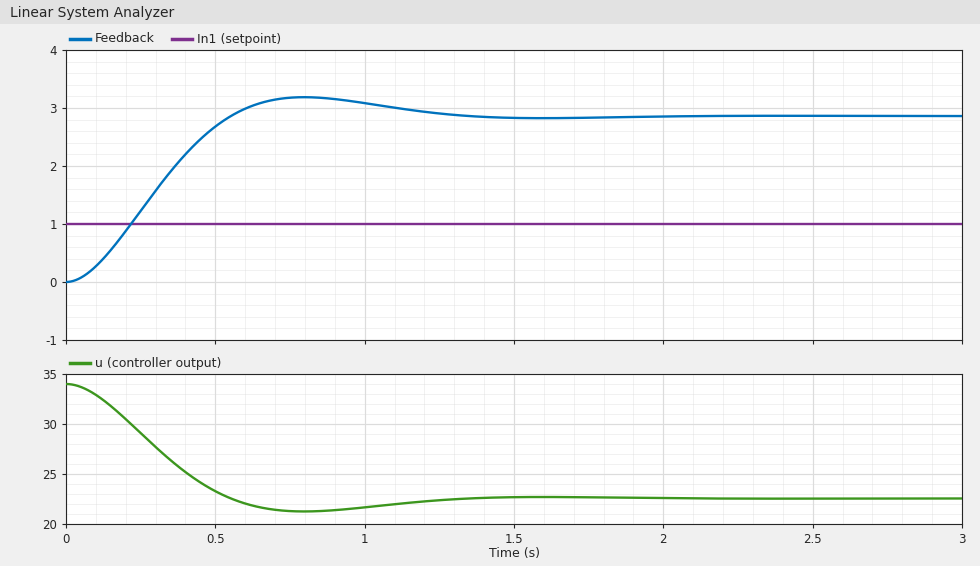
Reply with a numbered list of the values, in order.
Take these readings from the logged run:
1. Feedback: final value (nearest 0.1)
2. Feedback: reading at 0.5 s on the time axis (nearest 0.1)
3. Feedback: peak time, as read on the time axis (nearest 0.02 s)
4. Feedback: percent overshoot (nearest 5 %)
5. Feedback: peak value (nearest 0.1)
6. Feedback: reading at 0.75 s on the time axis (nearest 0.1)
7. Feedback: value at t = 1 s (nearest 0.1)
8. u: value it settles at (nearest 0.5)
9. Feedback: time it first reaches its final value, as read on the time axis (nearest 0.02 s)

1. 2.9
2. 2.7
3. 0.80 s
4. 10 %
5. 3.2
6. 3.2
7. 3.1
8. 22.5
9. 0.56 s
